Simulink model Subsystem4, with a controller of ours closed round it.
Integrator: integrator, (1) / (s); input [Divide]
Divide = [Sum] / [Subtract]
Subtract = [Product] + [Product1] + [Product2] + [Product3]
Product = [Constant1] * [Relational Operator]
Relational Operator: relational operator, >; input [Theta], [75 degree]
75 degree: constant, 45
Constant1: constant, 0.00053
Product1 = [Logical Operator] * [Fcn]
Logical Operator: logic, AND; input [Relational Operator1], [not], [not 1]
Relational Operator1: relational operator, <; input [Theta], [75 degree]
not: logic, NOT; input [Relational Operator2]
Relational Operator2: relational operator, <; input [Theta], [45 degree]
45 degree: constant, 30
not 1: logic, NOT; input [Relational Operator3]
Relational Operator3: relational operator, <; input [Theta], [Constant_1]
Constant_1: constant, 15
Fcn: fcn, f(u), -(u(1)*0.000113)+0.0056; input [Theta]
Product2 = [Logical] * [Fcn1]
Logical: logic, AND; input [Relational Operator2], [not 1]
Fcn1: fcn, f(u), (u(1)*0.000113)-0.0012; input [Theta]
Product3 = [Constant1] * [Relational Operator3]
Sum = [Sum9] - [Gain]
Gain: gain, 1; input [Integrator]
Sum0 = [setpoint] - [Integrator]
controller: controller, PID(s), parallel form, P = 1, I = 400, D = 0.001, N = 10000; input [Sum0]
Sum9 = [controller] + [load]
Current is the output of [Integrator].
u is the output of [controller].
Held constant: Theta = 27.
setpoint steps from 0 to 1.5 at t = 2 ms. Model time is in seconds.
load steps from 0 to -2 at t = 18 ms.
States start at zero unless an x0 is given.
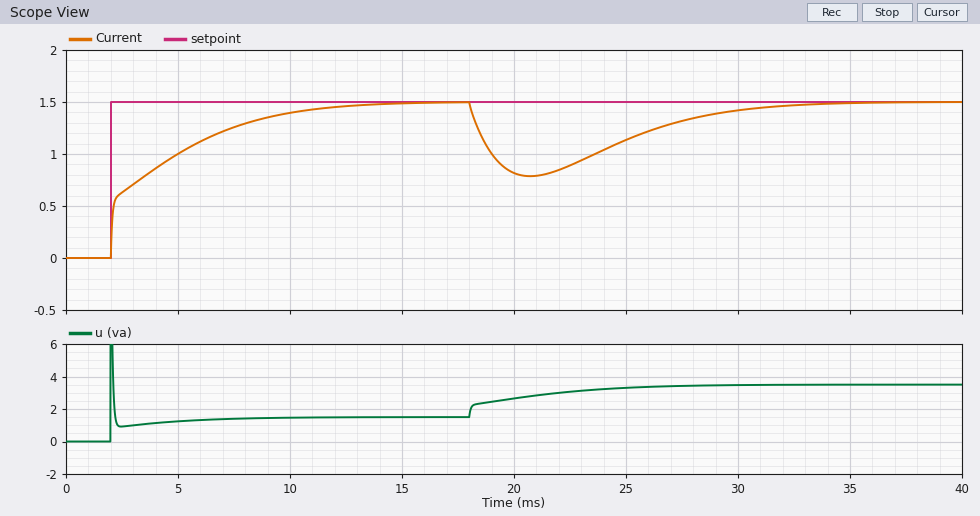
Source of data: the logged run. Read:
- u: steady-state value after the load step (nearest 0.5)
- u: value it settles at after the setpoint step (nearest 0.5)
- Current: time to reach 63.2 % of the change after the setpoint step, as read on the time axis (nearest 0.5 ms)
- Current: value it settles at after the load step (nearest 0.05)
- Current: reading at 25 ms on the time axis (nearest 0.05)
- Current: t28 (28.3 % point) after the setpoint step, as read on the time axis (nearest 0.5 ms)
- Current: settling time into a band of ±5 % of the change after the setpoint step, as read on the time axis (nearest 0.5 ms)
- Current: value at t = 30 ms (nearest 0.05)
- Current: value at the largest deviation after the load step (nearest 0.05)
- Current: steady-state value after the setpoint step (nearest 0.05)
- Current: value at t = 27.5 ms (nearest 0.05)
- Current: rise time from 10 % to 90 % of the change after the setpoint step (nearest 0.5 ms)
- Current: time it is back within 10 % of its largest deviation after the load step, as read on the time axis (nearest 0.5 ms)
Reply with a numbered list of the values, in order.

1. 3.5
2. 1.5
3. 4.5 ms
4. 1.50
5. 1.15
6. 2.0 ms
7. 11.0 ms
8. 1.40
9. 0.80
10. 1.50
11. 1.30
12. 7.0 ms
13. 30.5 ms
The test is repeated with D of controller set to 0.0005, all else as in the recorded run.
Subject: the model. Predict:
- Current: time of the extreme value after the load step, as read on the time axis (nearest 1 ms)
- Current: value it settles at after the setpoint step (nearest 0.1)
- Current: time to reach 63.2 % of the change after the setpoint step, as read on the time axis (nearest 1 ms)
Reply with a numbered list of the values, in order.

1. 20 ms
2. 1.5
3. 4 ms
